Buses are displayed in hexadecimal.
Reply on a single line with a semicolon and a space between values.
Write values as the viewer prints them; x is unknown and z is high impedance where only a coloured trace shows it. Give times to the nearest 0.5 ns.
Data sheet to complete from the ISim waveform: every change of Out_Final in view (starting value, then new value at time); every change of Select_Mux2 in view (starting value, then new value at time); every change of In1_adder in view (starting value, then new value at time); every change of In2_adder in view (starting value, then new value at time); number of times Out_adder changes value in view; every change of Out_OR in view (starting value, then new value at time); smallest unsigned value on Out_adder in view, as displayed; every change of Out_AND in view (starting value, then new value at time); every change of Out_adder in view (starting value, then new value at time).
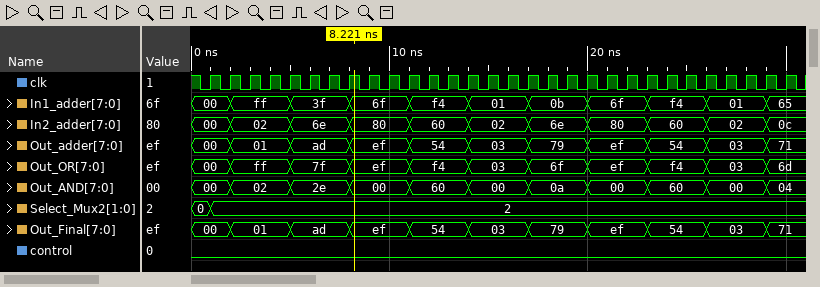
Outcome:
00, 01 at 2 ns, ad at 5 ns, ef at 8 ns, 54 at 11 ns, 03 at 14 ns, 79 at 17 ns, ef at 20 ns, 54 at 23 ns, 03 at 26 ns, 71 at 29 ns; 0, 2 at 1 ns; 00, ff at 2 ns, 3f at 5 ns, 6f at 8 ns, f4 at 11 ns, 01 at 14 ns, 0b at 17 ns, 6f at 20 ns, f4 at 23 ns, 01 at 26 ns, 65 at 29 ns; 00, 02 at 2 ns, 6e at 5 ns, 80 at 8 ns, 60 at 11 ns, 02 at 14 ns, 6e at 17 ns, 80 at 20 ns, 60 at 23 ns, 02 at 26 ns, 0c at 29 ns; 10; 00, ff at 2 ns, 7f at 5 ns, ef at 8 ns, f4 at 11 ns, 03 at 14 ns, 6f at 17 ns, ef at 20 ns, f4 at 23 ns, 03 at 26 ns, 6d at 29 ns; 00; 00, 02 at 2 ns, 2e at 5 ns, 00 at 8 ns, 60 at 11 ns, 00 at 14 ns, 0a at 17 ns, 00 at 20 ns, 60 at 23 ns, 00 at 26 ns, 04 at 29 ns; 00, 01 at 2 ns, ad at 5 ns, ef at 8 ns, 54 at 11 ns, 03 at 14 ns, 79 at 17 ns, ef at 20 ns, 54 at 23 ns, 03 at 26 ns, 71 at 29 ns
